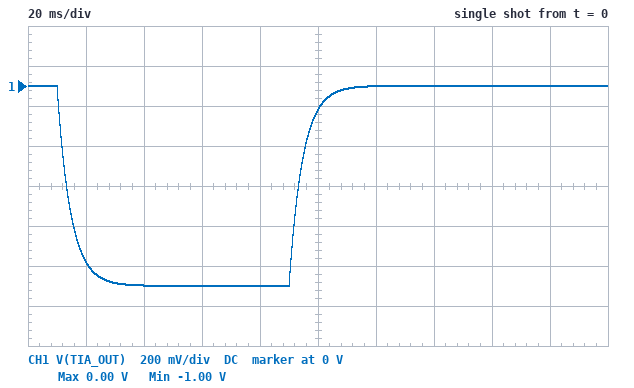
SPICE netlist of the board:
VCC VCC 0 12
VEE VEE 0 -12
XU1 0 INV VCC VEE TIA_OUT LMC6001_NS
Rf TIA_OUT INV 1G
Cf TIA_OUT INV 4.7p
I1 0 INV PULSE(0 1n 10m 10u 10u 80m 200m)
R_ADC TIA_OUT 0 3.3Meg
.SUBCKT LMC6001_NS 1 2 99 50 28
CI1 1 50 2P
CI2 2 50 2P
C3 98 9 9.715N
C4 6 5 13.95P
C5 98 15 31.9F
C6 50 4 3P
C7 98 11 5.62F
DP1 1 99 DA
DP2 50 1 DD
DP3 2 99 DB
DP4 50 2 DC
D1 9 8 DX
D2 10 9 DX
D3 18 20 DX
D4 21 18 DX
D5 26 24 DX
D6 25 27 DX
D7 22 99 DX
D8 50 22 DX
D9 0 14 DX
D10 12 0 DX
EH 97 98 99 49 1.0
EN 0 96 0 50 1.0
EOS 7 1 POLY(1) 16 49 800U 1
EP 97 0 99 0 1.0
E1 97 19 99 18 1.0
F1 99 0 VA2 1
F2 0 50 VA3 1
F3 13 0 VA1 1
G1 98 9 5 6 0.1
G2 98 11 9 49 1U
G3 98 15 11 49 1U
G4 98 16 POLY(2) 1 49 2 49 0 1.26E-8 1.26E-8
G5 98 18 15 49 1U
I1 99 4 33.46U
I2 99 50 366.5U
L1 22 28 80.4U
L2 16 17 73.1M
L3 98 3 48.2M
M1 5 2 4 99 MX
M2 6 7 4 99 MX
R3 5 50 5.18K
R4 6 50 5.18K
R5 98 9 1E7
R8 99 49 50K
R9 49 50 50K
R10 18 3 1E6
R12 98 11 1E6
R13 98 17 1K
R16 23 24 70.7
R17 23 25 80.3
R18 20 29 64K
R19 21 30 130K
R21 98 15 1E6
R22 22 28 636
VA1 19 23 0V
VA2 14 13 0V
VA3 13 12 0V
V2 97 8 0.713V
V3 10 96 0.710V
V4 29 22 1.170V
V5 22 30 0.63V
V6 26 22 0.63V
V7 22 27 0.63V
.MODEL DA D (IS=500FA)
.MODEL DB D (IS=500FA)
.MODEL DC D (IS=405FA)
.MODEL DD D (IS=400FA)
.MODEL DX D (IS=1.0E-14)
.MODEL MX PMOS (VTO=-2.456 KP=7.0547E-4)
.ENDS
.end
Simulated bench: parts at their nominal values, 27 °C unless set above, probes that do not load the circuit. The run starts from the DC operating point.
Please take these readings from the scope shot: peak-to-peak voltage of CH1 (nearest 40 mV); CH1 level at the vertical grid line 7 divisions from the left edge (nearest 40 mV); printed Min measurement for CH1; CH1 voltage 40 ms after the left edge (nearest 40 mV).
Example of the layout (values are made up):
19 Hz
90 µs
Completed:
1.00 V
0 V
-1.00 V
-1.00 V
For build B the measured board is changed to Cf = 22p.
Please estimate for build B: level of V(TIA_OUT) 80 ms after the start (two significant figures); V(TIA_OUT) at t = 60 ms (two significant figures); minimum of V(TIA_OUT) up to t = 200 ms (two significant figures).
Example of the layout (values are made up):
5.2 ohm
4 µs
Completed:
-960 mV
-900 mV
-970 mV
